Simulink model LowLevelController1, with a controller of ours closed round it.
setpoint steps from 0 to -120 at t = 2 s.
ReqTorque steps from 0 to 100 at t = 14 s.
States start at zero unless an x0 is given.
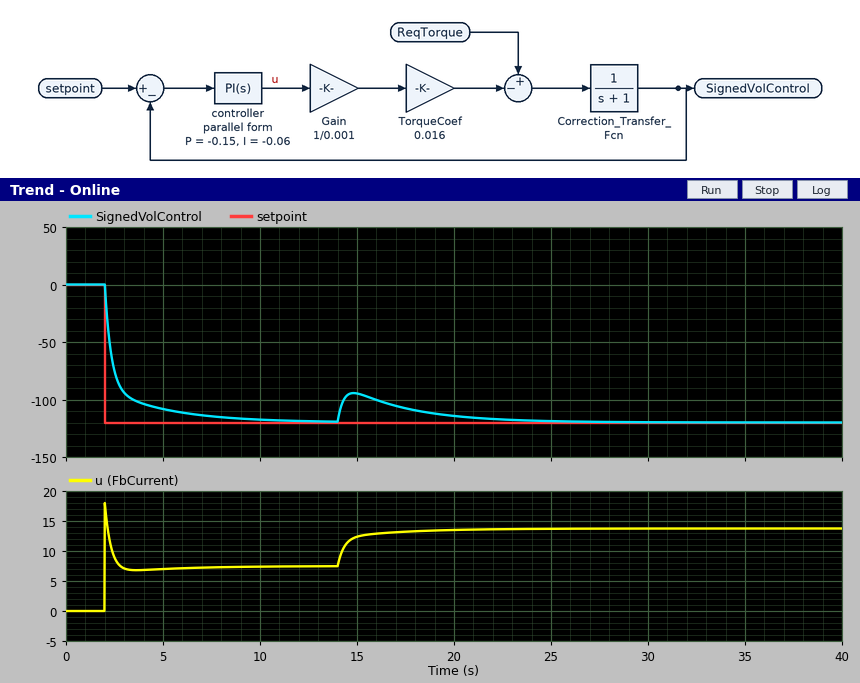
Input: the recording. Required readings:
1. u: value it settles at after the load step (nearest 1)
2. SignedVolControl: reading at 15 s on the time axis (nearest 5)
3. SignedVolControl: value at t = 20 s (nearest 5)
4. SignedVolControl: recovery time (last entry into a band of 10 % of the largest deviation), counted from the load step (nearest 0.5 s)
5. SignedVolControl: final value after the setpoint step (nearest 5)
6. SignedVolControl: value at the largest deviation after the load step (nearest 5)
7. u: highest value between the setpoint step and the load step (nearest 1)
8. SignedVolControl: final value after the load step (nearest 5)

14
-95
-115
8.5 s
-120
-95
18
-120
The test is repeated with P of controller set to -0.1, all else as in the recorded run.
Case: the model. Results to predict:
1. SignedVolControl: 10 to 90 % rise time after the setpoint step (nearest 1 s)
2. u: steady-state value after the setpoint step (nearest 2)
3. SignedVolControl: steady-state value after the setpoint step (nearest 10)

3 s
8
-120
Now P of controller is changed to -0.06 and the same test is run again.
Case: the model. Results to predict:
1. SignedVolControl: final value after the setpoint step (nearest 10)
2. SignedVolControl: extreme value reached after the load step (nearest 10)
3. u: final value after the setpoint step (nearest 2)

-120
-80
8
